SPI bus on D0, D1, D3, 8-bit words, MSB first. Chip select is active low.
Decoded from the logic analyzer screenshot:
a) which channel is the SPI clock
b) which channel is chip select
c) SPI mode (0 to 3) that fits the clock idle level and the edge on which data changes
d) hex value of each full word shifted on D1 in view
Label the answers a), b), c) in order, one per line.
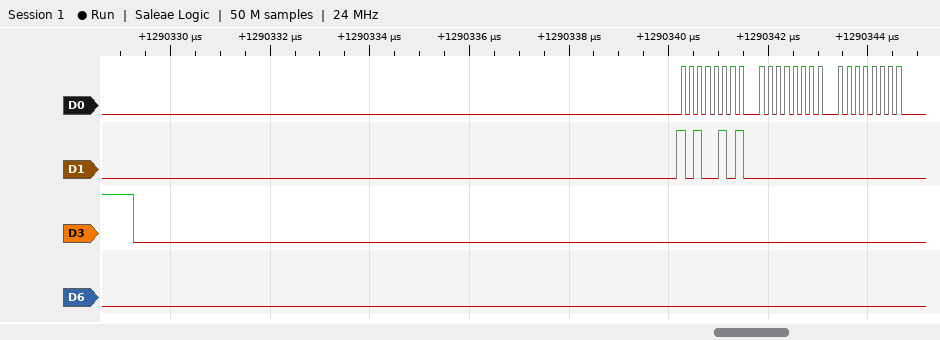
a) D0
b) D3
c) 0
d) A5, 00, 00
